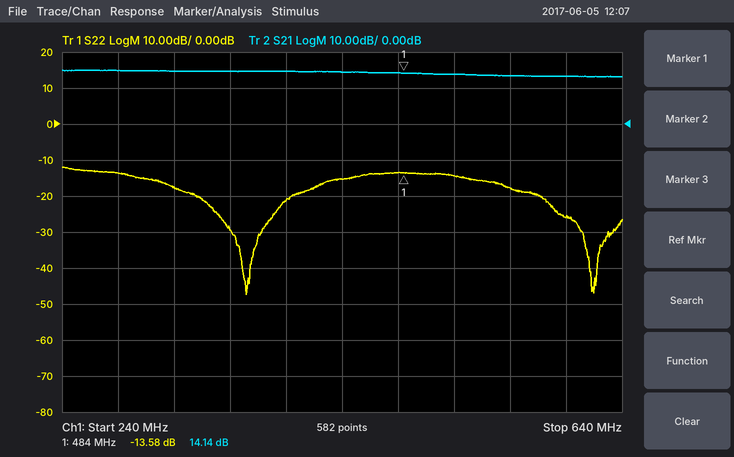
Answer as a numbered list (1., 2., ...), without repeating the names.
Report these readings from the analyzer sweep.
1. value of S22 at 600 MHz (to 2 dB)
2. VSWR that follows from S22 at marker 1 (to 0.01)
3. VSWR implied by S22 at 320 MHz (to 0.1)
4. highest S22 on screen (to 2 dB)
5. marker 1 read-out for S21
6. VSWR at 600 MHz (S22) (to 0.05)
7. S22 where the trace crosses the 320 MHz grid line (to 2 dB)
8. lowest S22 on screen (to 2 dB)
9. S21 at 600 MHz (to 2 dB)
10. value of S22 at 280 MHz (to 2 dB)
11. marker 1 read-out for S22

1. -26 dB
2. 1.53
3. 1.3
4. -12 dB
5. 14.14 dB
6. 1.10
7. -18 dB
8. -48 dB
9. 14 dB
10. -14 dB
11. -13.58 dB
